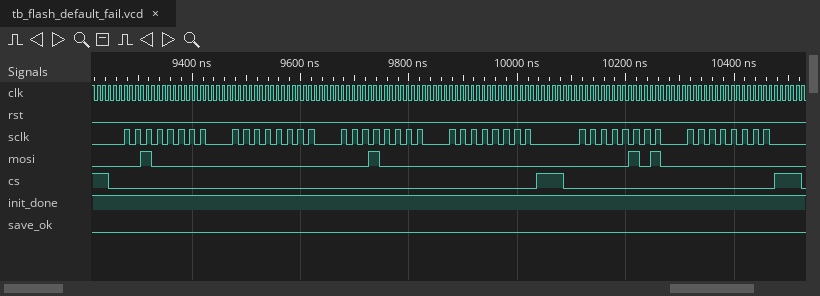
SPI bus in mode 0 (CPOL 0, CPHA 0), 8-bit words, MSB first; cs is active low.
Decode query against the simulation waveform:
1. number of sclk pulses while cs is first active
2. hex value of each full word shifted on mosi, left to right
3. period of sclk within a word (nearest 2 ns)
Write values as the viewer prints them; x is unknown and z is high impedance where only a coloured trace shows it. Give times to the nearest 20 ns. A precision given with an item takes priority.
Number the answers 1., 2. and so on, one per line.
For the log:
1. 32
2. 20, 00, 10, 00, 05, 00
3. 20 ns
